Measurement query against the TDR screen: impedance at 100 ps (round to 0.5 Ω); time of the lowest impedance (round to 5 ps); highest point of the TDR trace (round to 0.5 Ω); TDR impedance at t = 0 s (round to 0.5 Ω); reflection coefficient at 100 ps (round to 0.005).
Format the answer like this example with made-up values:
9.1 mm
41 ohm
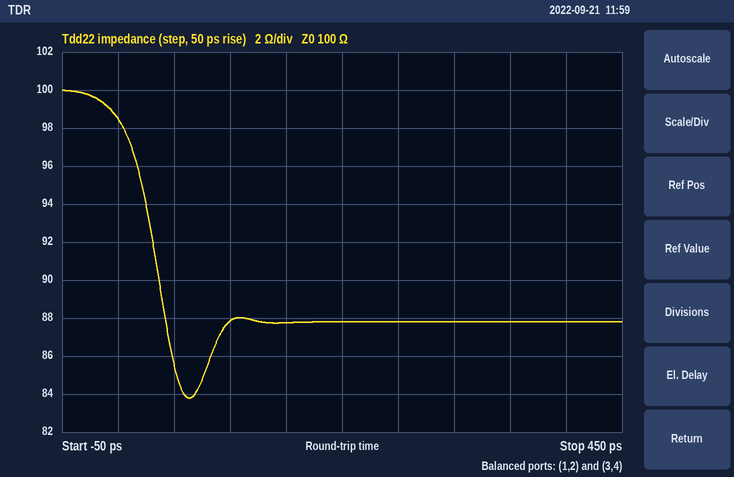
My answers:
88.0 Ω
65 ps
100.0 Ω
98.5 Ω
-0.065
